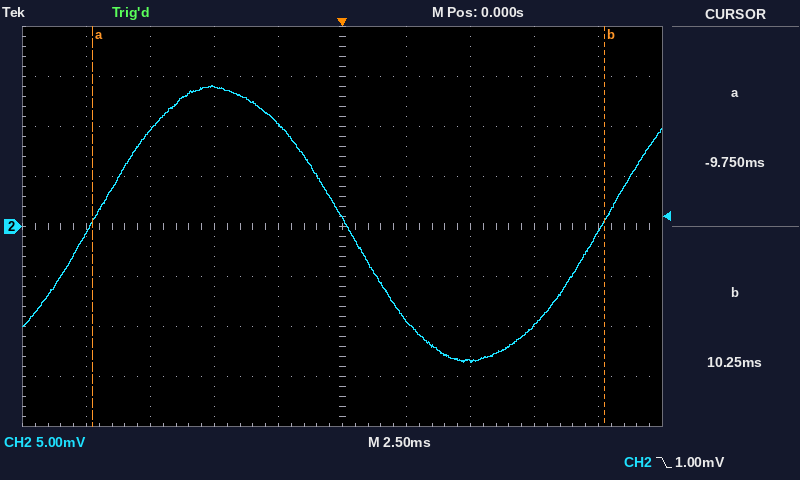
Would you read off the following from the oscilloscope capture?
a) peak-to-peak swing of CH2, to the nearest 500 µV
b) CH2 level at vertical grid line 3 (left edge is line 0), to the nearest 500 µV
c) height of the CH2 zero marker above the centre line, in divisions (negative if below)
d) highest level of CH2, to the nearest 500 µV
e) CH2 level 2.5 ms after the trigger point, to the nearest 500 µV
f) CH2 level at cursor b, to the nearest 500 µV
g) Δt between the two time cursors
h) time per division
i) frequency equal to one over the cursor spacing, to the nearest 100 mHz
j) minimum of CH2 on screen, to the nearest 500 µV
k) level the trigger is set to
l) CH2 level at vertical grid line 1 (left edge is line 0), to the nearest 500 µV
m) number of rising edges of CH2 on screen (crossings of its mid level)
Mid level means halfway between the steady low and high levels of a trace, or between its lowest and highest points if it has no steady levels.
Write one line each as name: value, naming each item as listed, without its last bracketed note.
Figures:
peak-to-peak swing of CH2, to the nearest 500 µV: 27.5 mV
CH2 level at vertical grid line 3 (left edge is line 0), to the nearest 500 µV: 14.0 mV
height of the CH2 zero marker above the centre line, in divisions: 0.0 div
highest level of CH2, to the nearest 500 µV: 14.0 mV
CH2 level 2.5 ms after the trigger point, to the nearest 500 µV: -9.5 mV
CH2 level at cursor b, to the nearest 500 µV: 500 µV
Δt between the two time cursors: 20.00 ms
time per division: 2.5 ms
frequency equal to one over the cursor spacing, to the nearest 100 mHz: 50.0 Hz
minimum of CH2 on screen, to the nearest 500 µV: -13.5 mV
level the trigger is set to: 1.00 mV
CH2 level at vertical grid line 1 (left edge is line 0), to the nearest 500 µV: -500 µV
number of rising edges of CH2 on screen: 2
